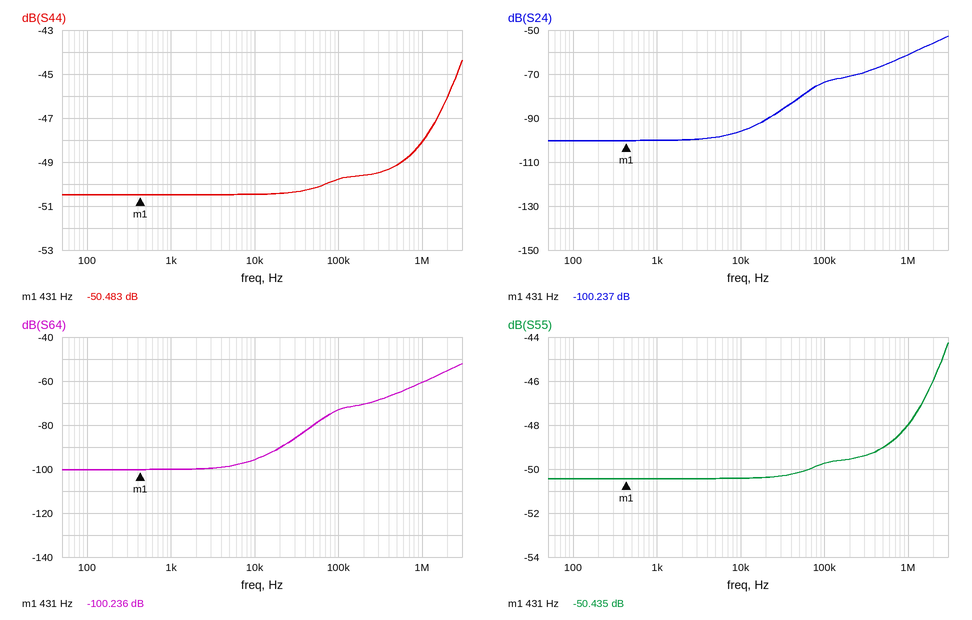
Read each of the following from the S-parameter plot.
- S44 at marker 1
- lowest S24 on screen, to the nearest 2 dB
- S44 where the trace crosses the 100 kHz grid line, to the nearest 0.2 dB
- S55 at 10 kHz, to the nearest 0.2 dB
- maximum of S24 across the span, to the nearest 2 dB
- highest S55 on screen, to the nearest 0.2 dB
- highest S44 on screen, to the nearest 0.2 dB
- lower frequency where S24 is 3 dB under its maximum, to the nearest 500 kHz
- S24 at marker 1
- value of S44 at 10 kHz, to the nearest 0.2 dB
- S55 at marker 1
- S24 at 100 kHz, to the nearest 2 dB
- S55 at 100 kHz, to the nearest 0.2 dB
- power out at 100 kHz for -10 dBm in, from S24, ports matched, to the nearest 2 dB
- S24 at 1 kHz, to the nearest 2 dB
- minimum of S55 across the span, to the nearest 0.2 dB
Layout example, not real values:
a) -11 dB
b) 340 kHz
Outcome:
a) -50.483 dB
b) -100 dB
c) -49.8 dB
d) -50.4 dB
e) -52 dB
f) -44.2 dB
g) -44.4 dB
h) 2.0 MHz
i) -100.237 dB
j) -50.4 dB
k) -50.435 dB
l) -74 dB
m) -49.8 dB
n) -84 dBm
o) -100 dB
p) -50.4 dB
